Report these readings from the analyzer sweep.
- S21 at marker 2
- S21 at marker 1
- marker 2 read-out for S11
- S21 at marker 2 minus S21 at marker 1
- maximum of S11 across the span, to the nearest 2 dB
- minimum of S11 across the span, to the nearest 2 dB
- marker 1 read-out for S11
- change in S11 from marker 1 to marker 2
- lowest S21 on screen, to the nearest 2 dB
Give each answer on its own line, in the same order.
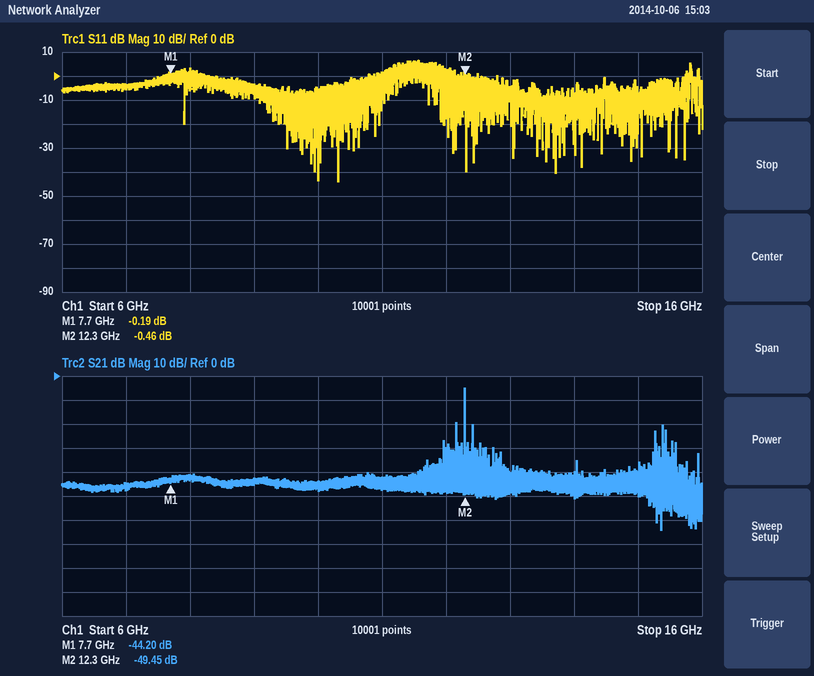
-49.45 dB
-44.20 dB
-0.46 dB
-5.25 dB
6 dB
-44 dB
-0.19 dB
-0.27 dB
-64 dB
